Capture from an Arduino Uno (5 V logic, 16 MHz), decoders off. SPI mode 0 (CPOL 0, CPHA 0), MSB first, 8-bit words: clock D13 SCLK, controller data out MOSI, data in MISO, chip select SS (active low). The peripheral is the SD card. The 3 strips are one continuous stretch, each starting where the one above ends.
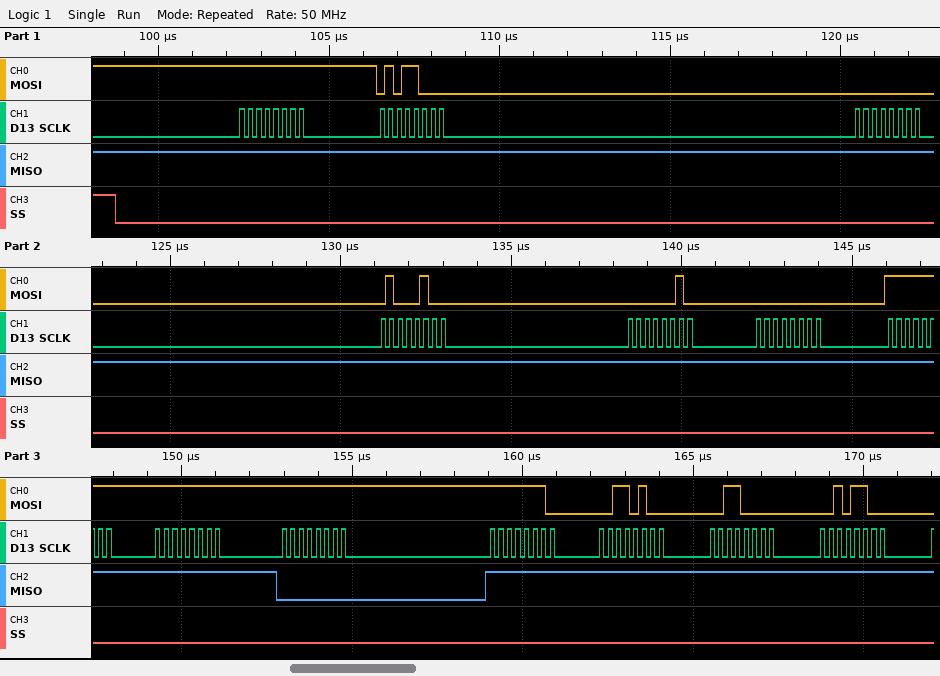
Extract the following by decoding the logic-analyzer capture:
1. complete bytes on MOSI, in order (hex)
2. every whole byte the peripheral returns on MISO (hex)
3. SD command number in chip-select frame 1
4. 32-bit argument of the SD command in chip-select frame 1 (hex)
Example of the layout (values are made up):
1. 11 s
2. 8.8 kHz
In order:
1. FF 58 00 44 02 00 FF FF FF FE 34 30 2C
2. FF FF FF FF FF FF FF FF 00 FF FF FF FF
3. CMD24
4. 0x00440200
